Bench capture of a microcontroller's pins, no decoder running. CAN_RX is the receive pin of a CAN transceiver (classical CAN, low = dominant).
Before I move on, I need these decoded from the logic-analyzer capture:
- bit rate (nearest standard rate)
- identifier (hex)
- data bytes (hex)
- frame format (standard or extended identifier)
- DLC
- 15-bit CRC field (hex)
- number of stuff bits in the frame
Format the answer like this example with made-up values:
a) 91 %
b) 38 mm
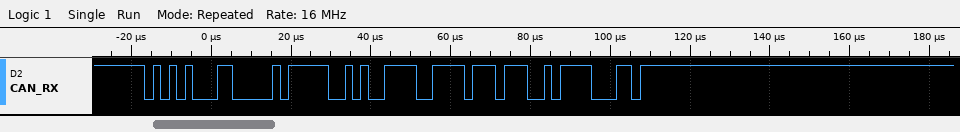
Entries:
a) 500 kbit/s
b) 0x546
c) EA 79 EE
d) standard
e) 3
f) 0x72F1
g) 2
